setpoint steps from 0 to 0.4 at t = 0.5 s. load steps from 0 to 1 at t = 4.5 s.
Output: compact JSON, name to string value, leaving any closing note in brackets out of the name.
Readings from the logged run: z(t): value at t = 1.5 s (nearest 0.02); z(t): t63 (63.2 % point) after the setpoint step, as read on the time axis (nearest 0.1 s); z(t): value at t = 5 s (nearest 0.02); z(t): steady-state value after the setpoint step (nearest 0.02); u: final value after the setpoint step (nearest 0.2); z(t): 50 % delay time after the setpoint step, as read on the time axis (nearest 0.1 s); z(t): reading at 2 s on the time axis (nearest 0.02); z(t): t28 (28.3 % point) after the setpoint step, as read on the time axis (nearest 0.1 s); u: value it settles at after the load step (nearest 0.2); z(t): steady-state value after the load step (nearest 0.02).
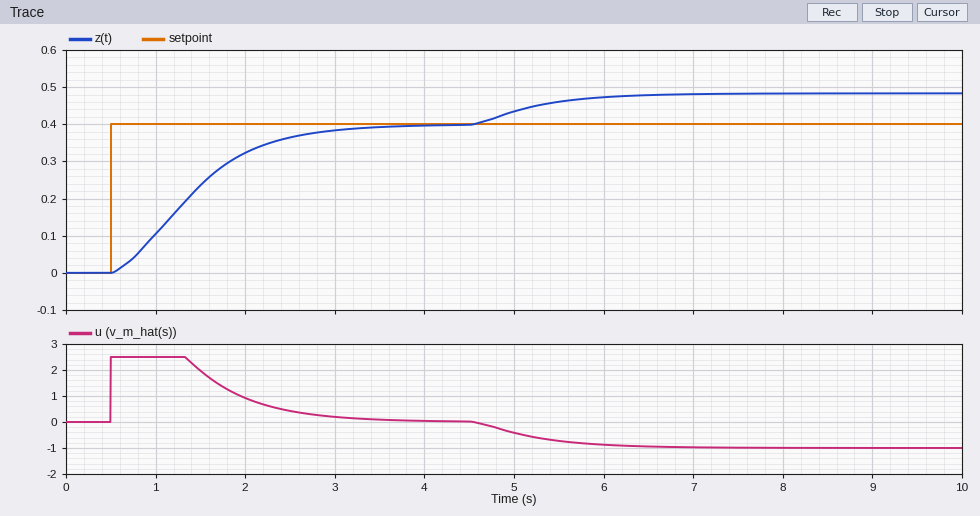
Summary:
{"z(t): value at t = 1.5 s": "0.24", "z(t): t63 (63.2 % point) after the setpoint step, as read on the time axis": "1.6 s", "z(t): value at t = 5 s": "0.44", "z(t): steady-state value after the setpoint step": "0.40", "u: final value after the setpoint step": "0.0", "z(t): 50 % delay time after the setpoint step, as read on the time axis": "1.4 s", "z(t): reading at 2 s on the time axis": "0.32", "z(t): t28 (28.3 % point) after the setpoint step, as read on the time axis": "1.0 s", "u: value it settles at after the load step": "-1.0", "z(t): steady-state value after the load step": "0.48"}
